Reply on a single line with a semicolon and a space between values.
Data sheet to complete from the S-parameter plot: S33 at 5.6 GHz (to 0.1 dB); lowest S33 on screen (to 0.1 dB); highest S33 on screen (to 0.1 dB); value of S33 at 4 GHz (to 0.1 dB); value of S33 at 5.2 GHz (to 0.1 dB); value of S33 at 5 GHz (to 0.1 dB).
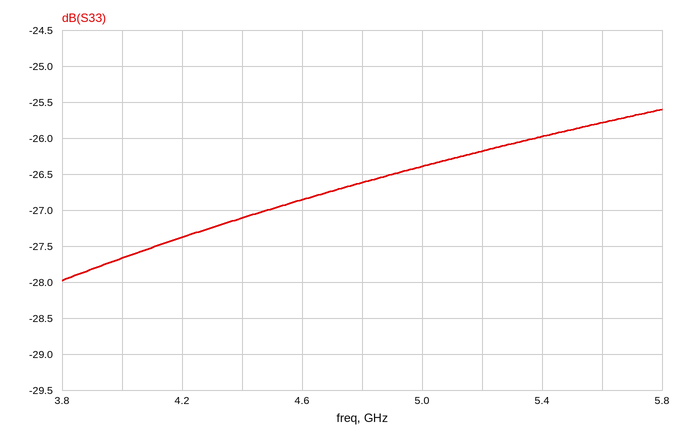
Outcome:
-25.8 dB; -28.0 dB; -25.6 dB; -27.7 dB; -26.2 dB; -26.4 dB
